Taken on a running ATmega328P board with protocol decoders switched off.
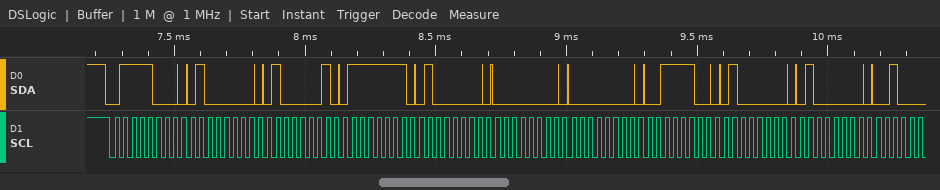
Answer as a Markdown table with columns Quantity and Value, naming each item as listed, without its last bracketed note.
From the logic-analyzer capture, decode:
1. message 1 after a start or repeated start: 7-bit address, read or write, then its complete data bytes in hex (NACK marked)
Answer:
| Quantity | Value |
|---|---|
| message 1 after a start or repeated start: 7-bit address, read or write, then its complete data bytes in hex | 0x3C write: 40 41 7F 40 00 00 3C 40 40 |
